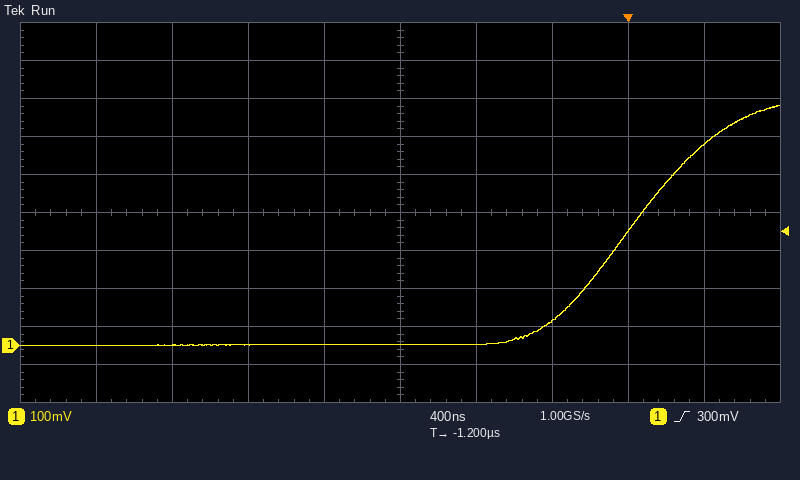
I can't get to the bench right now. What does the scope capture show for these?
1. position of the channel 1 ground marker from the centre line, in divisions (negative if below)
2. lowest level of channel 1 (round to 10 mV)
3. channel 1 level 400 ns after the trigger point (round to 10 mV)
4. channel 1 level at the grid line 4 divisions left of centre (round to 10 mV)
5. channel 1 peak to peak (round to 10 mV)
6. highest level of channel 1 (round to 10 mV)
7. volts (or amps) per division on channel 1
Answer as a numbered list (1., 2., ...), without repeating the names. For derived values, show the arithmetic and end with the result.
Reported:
1. -3.5 div
2. 0 mV
3. 530 mV
4. 0 mV
5. 630 mV − (0 mV) = 630 mV
6. 630 mV
7. 100 mV
